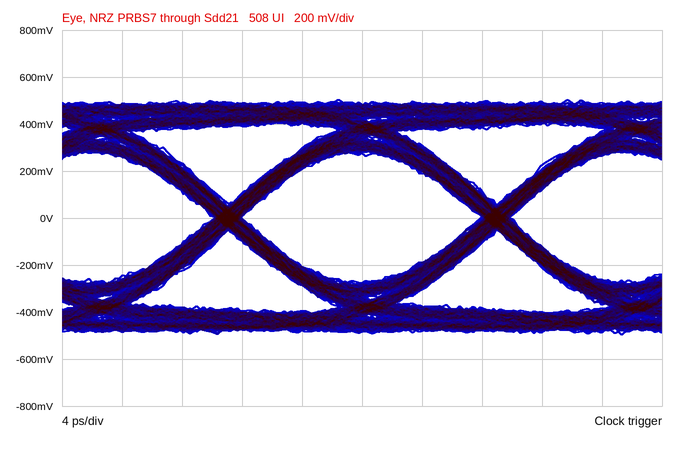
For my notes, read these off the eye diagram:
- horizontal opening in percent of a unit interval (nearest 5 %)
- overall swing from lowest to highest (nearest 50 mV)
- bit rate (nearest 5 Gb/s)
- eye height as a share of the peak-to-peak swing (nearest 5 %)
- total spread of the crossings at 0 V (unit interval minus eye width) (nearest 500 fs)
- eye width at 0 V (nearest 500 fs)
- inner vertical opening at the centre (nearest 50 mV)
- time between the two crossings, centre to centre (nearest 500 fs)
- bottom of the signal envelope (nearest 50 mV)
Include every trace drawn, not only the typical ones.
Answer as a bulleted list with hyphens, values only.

- 90 %
- 1.00 V
- 55 Gb/s
- 55 %
- 2.0 ps
- 16.0 ps
- 550 mV
- 18.0 ps
- -500 mV
